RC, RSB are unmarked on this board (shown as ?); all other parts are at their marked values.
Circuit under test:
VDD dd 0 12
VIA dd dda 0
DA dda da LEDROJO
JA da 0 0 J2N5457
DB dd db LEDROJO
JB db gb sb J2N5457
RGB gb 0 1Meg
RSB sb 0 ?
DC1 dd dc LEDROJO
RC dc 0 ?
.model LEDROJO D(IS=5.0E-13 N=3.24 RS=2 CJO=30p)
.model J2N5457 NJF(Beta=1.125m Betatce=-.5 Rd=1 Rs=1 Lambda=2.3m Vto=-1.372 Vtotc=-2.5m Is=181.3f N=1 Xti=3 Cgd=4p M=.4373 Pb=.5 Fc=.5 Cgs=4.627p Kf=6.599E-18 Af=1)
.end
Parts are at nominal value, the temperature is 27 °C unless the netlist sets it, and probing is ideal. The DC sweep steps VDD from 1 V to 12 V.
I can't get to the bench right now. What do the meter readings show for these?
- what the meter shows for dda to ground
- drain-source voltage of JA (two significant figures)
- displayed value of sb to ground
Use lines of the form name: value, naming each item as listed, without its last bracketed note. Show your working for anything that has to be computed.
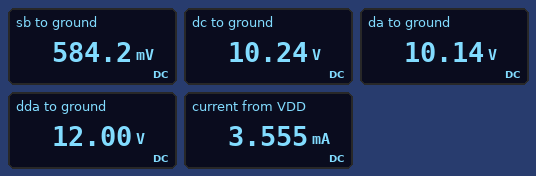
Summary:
what the meter shows for dda to ground: 12.00 V
drain-source voltage of JA: 10.14 V = 10 V
displayed value of sb to ground: 584.2 mV
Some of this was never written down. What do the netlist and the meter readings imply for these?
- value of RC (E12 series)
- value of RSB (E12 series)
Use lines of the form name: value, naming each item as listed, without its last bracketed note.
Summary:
value of RC: 15 kΩ
value of RSB: 820 Ω
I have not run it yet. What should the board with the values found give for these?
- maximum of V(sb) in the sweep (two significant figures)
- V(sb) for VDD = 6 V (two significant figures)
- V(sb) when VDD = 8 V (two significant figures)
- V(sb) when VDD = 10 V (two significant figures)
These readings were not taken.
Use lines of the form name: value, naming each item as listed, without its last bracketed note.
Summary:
maximum of V(sb) in the sweep: 580 mV
V(sb) for VDD = 6 V: 580 mV
V(sb) when VDD = 8 V: 580 mV
V(sb) when VDD = 10 V: 580 mV
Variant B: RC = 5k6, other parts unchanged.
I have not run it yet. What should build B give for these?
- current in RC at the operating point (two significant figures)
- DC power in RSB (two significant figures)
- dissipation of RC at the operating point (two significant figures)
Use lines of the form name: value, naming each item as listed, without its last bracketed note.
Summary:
current in RC at the operating point: 1.8 mA
DC power in RSB: 420 µW
dissipation of RC at the operating point: 18 mW
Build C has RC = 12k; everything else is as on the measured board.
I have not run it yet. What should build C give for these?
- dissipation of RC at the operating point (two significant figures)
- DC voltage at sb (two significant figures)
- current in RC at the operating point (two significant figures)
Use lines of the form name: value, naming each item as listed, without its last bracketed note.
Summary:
dissipation of RC at the operating point: 8.7 mW
DC voltage at sb: 580 mV
current in RC at the operating point: 850 µA
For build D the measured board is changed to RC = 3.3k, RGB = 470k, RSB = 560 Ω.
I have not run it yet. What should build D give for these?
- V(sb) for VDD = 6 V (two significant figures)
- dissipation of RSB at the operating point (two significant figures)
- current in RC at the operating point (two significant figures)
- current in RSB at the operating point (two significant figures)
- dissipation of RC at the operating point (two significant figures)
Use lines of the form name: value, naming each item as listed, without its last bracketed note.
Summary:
V(sb) for VDD = 6 V: 490 mV
dissipation of RSB at the operating point: 440 µW
current in RC at the operating point: 3.1 mA
current in RSB at the operating point: 880 µA
dissipation of RC at the operating point: 31 mW
